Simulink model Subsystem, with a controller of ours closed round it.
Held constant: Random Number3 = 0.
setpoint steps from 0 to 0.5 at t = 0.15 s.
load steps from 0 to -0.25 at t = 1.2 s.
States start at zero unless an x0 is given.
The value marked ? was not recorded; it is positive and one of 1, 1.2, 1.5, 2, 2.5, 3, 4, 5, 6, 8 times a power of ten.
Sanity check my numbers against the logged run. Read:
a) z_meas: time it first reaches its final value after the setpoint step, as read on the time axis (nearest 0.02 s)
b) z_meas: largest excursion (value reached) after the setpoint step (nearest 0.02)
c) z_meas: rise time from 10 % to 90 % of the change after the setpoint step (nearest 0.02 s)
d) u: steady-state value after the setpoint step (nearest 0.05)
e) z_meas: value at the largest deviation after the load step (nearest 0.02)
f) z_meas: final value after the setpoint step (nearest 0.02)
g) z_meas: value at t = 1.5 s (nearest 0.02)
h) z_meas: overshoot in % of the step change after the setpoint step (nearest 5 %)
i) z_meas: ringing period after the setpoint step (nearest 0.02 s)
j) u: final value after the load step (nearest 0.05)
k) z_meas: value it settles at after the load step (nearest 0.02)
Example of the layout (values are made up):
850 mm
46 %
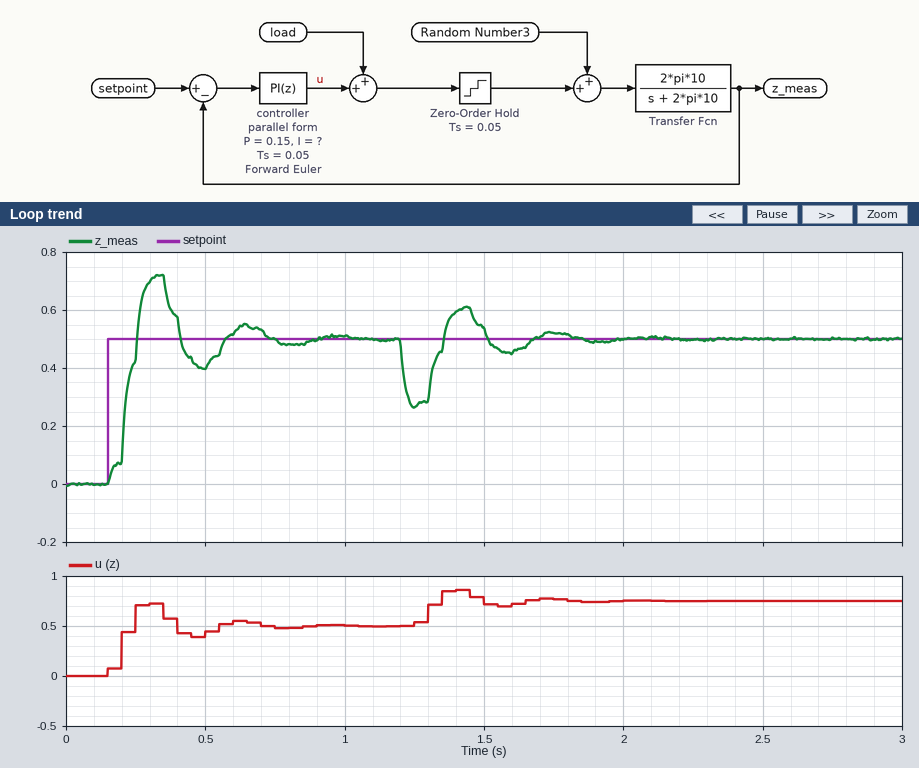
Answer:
0.26 s
0.72
0.08 s
0.50
0.26
0.50
0.54
45 %
0.30 s
0.75
0.50
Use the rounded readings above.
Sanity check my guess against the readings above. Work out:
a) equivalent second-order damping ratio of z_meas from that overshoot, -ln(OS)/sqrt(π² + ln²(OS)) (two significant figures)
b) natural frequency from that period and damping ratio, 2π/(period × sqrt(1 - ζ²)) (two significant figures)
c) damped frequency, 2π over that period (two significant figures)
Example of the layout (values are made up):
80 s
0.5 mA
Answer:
0.25
22 rad/s
21 rad/s
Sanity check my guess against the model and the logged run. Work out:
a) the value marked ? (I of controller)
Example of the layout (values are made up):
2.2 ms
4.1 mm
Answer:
15
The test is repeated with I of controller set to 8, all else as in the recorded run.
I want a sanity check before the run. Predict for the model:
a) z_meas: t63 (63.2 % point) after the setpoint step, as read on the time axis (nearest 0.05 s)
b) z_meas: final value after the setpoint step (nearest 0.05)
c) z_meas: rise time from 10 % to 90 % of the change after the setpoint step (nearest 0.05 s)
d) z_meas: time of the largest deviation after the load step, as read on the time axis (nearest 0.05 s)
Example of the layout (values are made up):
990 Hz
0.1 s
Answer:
0.25 s
0.50
0.15 s
1.25 s
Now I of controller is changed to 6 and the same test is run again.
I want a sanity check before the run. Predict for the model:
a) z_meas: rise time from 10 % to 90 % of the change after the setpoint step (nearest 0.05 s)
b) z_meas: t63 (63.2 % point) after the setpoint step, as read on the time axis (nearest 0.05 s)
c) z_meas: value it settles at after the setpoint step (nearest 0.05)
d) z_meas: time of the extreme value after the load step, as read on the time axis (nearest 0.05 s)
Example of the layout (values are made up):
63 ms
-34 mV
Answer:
0.25 s
0.30 s
0.50
1.25 s
